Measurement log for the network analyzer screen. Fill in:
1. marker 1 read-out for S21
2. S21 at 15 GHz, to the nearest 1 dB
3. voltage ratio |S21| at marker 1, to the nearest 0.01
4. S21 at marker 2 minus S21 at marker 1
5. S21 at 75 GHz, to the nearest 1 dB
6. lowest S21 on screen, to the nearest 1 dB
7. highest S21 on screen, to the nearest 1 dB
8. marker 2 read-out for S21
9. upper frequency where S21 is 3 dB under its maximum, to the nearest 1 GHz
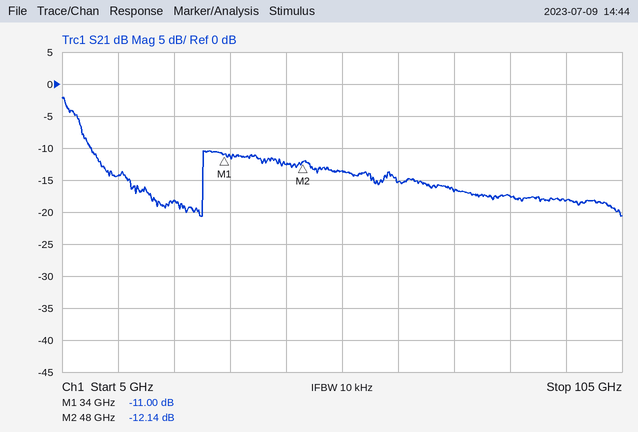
-11.00 dB
-14 dB
0.28
-1.14 dB
-17 dB
-21 dB
-2 dB
-12.14 dB
8 GHz
